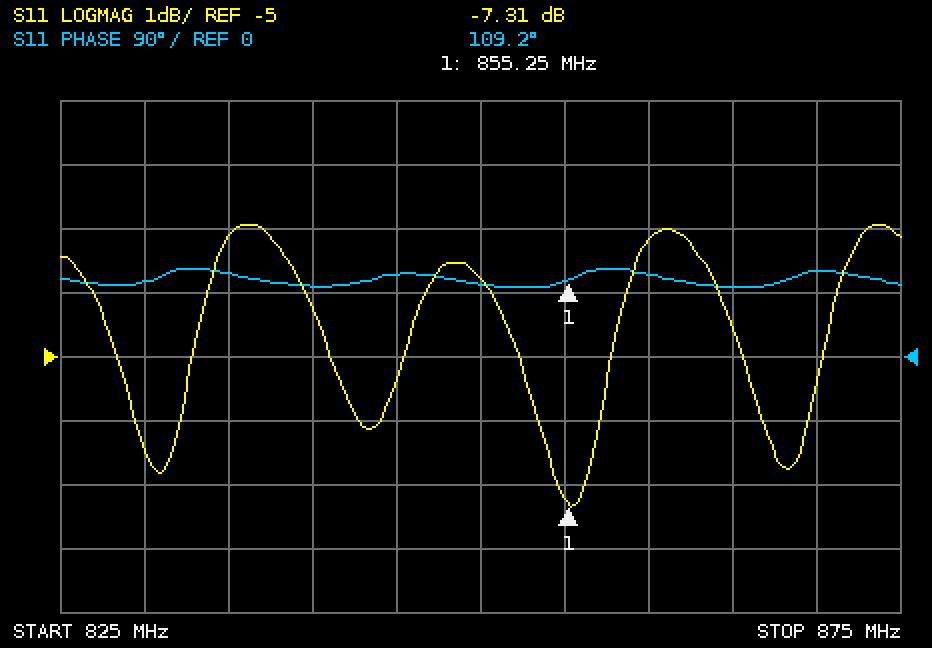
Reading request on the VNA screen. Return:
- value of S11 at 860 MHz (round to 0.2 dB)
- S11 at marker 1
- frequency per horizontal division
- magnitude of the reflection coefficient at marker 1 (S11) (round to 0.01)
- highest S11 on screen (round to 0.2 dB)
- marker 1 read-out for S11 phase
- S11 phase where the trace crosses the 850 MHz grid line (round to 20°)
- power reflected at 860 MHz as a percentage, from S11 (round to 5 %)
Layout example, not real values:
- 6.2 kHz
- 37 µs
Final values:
- -3.2 dB
- -7.31 dB
- 5 MHz
- 0.43
- -3.0 dB
- 109.2°
- 100°
- 50 %
